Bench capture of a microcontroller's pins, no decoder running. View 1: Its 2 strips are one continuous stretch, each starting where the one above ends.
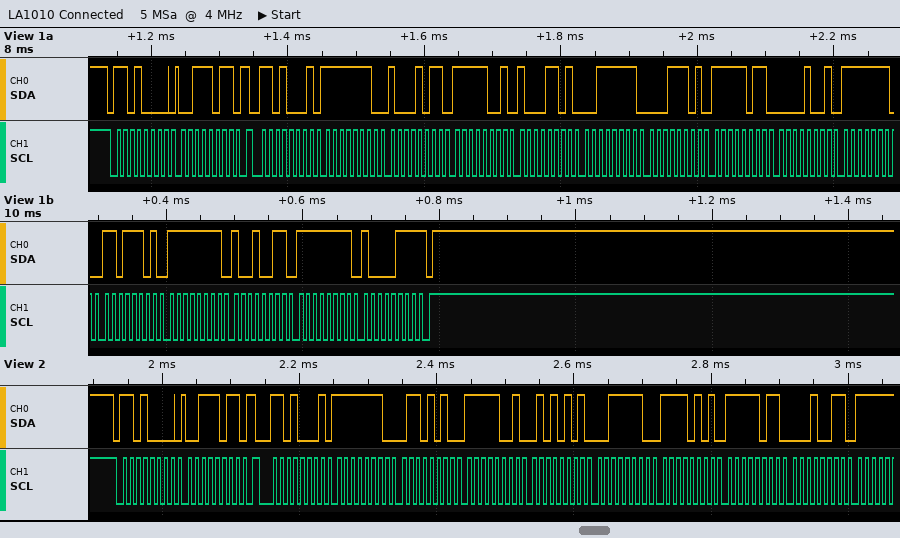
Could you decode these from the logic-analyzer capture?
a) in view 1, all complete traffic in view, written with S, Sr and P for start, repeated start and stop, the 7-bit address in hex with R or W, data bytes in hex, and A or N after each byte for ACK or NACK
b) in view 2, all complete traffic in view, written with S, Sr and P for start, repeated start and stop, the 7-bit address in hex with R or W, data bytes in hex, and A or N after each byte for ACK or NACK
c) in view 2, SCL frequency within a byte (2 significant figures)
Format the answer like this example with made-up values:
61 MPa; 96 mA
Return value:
S 68W A 3B A Sr 68R A FE A 8B A F9 A 8D A 3F A 1D A FB A 09 A FE A DD A FF A 93 A FF A 87 N P; S 68W A 3B A Sr 68R A FE A 6A A F9 A 55 A 3E A F5 A FB A 13 A; 100 kHz
